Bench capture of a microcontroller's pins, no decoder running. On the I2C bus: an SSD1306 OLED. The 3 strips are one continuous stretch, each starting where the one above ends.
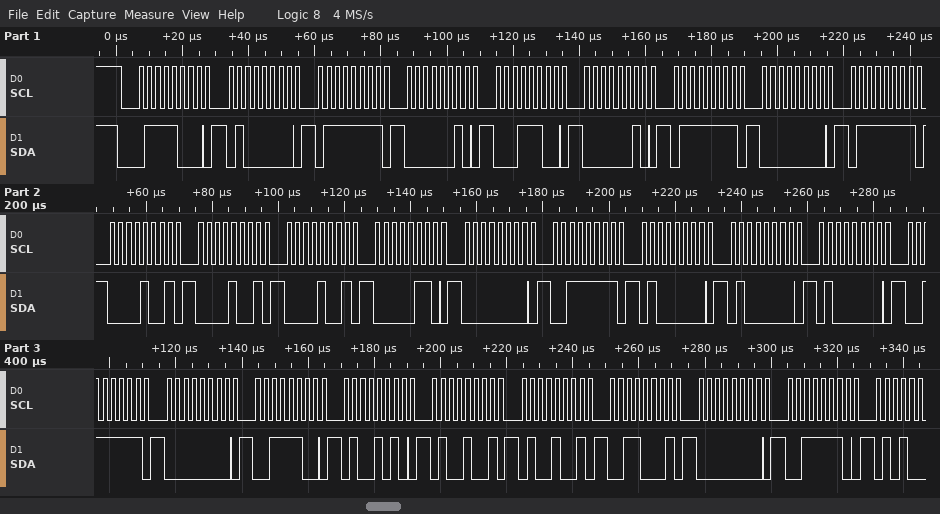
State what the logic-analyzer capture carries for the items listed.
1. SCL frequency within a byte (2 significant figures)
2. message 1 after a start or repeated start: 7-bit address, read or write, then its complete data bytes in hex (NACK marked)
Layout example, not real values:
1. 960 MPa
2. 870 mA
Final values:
1. 400 kHz
2. 0x3C write: 40 7F 02 1C 02 7F 00 7F 09 09 09 06 00 3F 40 40 40 3F 00 3C 4A 49 49 31 00 3E
